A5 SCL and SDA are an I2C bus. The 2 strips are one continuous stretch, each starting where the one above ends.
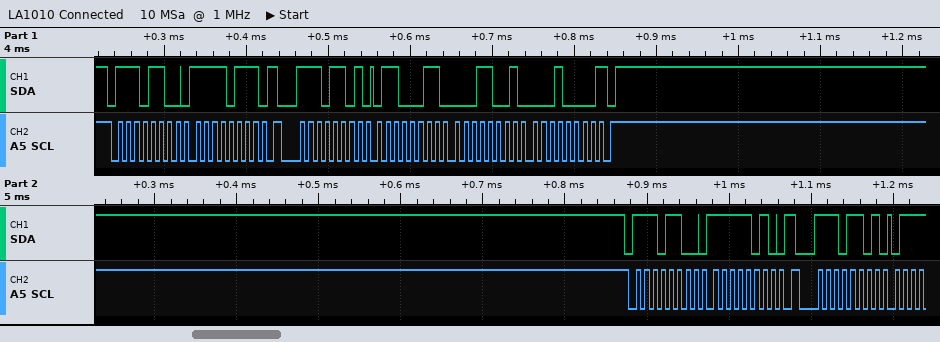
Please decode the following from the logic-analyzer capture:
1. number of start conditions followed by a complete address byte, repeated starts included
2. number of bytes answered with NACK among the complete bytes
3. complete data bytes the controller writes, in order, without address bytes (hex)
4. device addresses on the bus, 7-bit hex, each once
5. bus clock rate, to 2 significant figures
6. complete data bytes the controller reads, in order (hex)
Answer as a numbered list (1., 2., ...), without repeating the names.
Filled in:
1. 4
2. 1
3. F7 FA
4. 0x76
5. 100 kHz
6. 63 19 10
